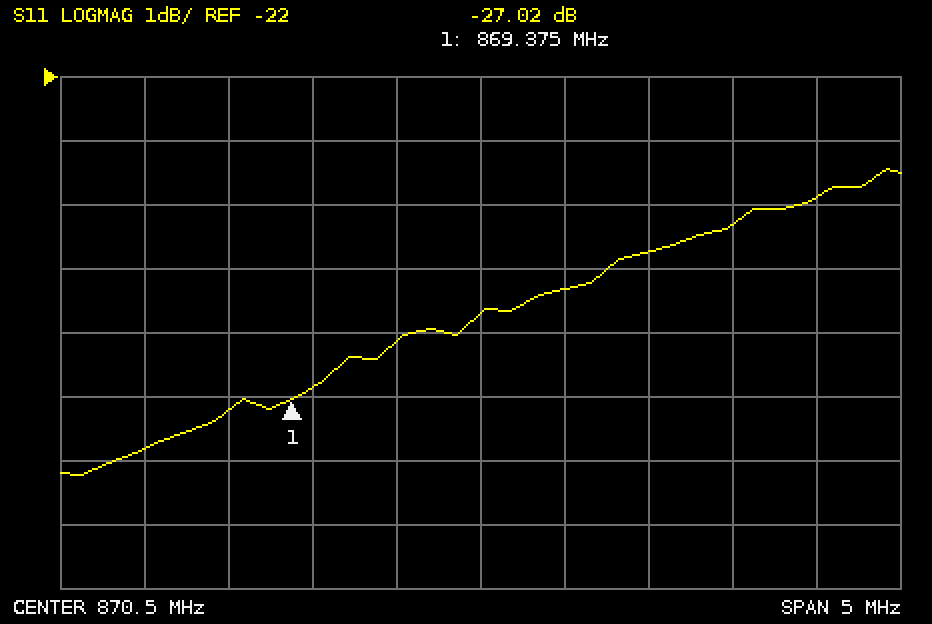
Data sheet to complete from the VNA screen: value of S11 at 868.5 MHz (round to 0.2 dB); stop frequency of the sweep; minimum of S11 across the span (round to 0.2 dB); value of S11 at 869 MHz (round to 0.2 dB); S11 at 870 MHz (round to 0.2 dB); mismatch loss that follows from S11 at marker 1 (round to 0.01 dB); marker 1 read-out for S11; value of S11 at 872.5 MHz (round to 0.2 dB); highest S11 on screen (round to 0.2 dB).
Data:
-27.8 dB
873 MHz
-28.2 dB
-27.2 dB
-26.2 dB
0.01 dB
-27.02 dB
-23.8 dB
-23.4 dB
